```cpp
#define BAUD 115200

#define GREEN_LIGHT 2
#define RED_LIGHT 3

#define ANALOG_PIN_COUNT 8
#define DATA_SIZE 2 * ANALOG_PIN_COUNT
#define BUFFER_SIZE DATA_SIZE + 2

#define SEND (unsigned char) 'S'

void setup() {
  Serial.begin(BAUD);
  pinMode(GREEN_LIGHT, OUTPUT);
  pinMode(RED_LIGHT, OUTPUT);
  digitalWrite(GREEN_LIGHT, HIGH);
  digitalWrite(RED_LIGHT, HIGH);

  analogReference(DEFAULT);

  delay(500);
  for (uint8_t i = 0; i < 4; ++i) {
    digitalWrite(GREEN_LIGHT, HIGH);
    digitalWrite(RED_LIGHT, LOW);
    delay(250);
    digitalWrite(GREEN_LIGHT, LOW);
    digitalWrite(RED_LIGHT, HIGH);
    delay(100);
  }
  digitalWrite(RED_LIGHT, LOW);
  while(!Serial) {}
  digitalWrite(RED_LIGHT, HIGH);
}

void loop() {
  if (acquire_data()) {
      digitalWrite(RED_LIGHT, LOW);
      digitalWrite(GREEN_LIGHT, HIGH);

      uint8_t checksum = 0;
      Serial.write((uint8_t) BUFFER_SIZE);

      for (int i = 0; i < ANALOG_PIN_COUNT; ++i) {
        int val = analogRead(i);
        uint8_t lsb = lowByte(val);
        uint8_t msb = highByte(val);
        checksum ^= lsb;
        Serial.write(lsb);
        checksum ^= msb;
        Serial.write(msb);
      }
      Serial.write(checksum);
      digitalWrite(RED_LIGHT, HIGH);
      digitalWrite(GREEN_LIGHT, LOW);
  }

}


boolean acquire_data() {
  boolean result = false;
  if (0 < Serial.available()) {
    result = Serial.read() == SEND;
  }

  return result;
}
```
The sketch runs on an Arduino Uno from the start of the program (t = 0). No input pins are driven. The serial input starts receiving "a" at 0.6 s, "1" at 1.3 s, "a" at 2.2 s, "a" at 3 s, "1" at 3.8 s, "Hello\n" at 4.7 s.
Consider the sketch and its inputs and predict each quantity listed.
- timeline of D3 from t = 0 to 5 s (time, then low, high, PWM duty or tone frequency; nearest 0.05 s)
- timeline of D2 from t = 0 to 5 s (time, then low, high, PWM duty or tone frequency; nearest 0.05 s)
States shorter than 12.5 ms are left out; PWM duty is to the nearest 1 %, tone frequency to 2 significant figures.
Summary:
0 s high; 0.5 s low; 0.75 s high; 0.85 s low; 1.1 s high; 1.2 s low; 1.45 s high; 1.55 s low; 1.8 s high
0 s high; 0.75 s low; 0.85 s high; 1.1 s low; 1.2 s high; 1.45 s low; 1.55 s high; 1.8 s low
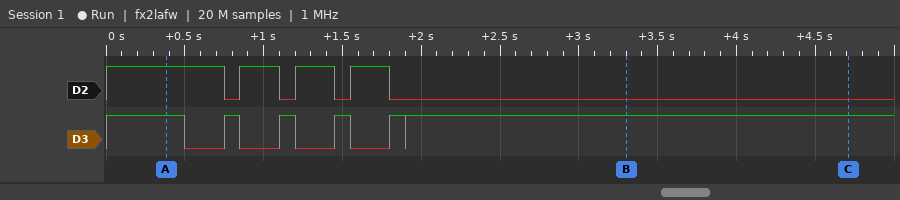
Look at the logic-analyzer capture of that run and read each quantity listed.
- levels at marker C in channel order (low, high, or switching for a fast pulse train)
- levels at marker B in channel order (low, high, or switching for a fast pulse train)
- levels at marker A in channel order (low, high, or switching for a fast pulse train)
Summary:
D2 low, D3 high
D2 low, D3 high
D2 high, D3 high
